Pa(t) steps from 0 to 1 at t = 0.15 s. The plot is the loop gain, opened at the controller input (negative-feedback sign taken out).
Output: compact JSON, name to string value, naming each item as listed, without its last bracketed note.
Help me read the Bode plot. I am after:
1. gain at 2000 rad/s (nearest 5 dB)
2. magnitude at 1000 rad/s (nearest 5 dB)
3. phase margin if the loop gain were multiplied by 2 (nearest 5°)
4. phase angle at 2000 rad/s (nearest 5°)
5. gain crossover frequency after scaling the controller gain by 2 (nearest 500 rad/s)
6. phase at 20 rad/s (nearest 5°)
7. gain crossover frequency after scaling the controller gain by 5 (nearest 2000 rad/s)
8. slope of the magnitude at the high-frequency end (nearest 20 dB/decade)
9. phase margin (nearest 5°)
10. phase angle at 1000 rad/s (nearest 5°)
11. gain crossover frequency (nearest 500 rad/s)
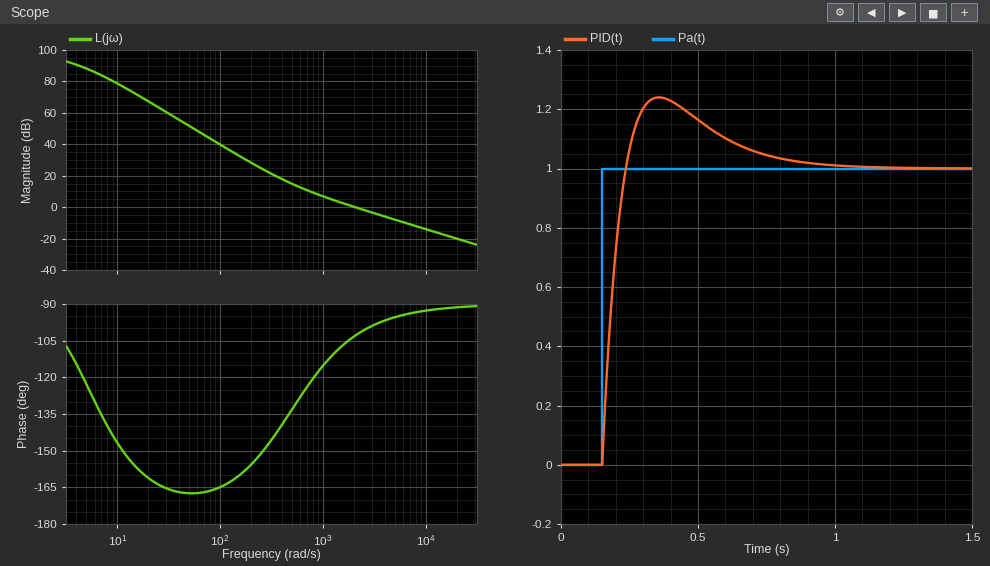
{"gain at 2000 rad/s": "0 dB", "magnitude at 1000 rad/s": "5 dB", "phase margin if the loop gain were multiplied by 2": "85°", "phase angle at 2000 rad/s": "-105°", "gain crossover frequency after scaling the controller gain by 2": "4000 rad/s", "phase at 20 rad/s": "-160°", "gain crossover frequency after scaling the controller gain by 5": "10000 rad/s", "slope of the magnitude at the high-frequency end": "-20 dB/decade", "phase margin": "75°", "phase angle at 1000 rad/s": "-115°", "gain crossover frequency": "2000 rad/s"}
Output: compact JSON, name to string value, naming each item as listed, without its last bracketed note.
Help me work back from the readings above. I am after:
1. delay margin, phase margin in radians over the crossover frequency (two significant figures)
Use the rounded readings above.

{"delay margin, phase margin in radians over the crossover frequency": "0.00065 s"}
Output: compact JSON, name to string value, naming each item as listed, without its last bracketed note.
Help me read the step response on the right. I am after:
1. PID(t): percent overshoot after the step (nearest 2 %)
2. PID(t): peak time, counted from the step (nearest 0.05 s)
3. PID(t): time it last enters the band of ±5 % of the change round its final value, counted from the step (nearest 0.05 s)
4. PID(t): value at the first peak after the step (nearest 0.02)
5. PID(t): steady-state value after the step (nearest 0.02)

{"PID(t): percent overshoot after the step": "24 %", "PID(t): peak time, counted from the step": "0.20 s", "PID(t): time it last enters the band of ±5 % of the change round its final value, counted from the step": "0.60 s", "PID(t): value at the first peak after the step": "1.24", "PID(t): steady-state value after the step": "1.00"}
